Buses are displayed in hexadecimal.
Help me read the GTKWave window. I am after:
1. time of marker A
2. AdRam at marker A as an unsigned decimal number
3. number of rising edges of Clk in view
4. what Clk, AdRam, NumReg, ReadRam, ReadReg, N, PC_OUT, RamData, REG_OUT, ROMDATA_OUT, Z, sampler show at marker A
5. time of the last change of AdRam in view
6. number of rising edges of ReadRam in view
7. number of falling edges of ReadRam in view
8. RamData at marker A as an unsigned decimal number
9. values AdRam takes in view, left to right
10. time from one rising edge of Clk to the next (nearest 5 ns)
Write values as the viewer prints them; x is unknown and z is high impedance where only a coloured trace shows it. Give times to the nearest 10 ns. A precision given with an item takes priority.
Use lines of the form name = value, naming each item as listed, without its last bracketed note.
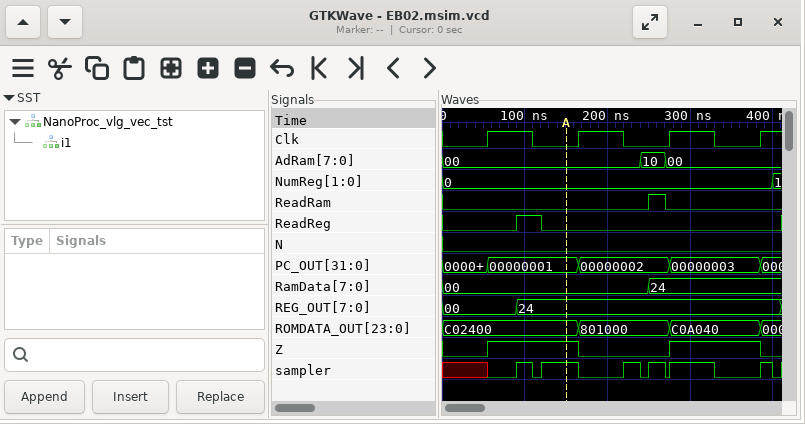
time of marker A = 150 ns
AdRam at marker A as an unsigned decimal number = 0
number of rising edges of Clk in view = 4
what Clk, AdRam, NumReg, ReadRam, ReadReg, N, PC_OUT, RamData, REG_OUT, ROMDATA_OUT, Z, sampler show at marker A = Clk=0, AdRam=00, NumReg=0, ReadRam=0, ReadReg=0, N=0, PC_OUT=00000001, RamData=00, REG_OUT=24, ROMDATA_OUT=C02400, Z=1, sampler=1
time of the last change of AdRam in view = 270 ns
number of rising edges of ReadRam in view = 1
number of falling edges of ReadRam in view = 1
RamData at marker A as an unsigned decimal number = 0
values AdRam takes in view, left to right = 00, 10, 00
time from one rising edge of Clk to the next = 110 ns
